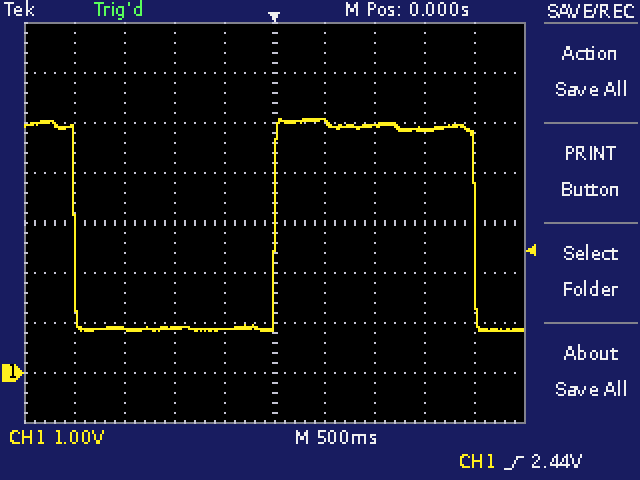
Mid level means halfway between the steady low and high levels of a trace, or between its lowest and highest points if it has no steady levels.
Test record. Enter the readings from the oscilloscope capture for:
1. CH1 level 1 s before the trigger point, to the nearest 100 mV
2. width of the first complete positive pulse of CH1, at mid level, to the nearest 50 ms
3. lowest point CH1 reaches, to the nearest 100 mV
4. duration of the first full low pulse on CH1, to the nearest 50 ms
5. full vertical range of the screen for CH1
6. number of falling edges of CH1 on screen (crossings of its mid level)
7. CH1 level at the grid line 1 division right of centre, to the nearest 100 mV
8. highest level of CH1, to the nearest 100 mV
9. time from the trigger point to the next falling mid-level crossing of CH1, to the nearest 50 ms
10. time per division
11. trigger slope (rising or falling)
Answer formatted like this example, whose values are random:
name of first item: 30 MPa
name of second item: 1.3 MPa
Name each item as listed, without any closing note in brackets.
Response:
CH1 level 1 s before the trigger point, to the nearest 100 mV: 900 mV
width of the first complete positive pulse of CH1, at mid level, to the nearest 50 ms: 2.00 s
lowest point CH1 reaches, to the nearest 100 mV: 800 mV
duration of the first full low pulse on CH1, to the nearest 50 ms: 2.00 s
full vertical range of the screen for CH1: 8 V
number of falling edges of CH1 on screen: 2
CH1 level at the grid line 1 division right of centre, to the nearest 100 mV: 5.0 V
highest level of CH1, to the nearest 100 mV: 5.1 V
time from the trigger point to the next falling mid-level crossing of CH1, to the nearest 50 ms: 2.00 s
time per division: 500 ms
trigger slope: rising
